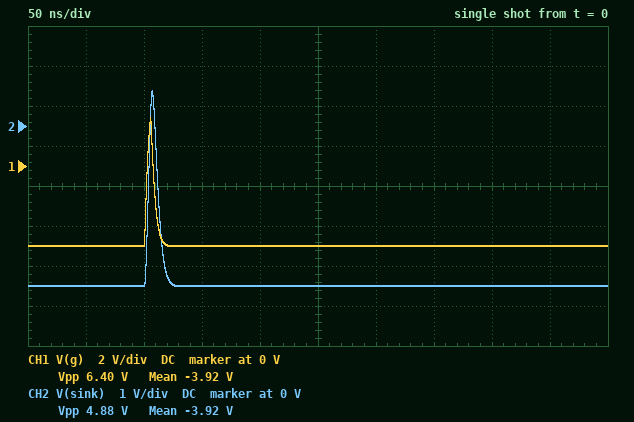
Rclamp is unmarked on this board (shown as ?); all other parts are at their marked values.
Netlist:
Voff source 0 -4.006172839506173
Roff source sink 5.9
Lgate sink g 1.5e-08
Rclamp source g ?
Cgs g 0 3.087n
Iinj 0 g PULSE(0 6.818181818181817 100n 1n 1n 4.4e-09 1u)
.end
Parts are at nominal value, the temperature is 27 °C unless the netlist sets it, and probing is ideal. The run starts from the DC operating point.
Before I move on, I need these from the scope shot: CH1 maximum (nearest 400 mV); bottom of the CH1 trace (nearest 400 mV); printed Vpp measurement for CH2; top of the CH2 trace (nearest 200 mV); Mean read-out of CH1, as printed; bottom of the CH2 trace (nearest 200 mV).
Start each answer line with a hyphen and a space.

- 2.4 V
- -4.0 V
- 4.88 V
- 800 mV
- -3.92 V
- -4.0 V
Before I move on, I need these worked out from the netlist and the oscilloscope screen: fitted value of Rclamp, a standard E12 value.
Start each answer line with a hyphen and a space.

- 1.5 Ω
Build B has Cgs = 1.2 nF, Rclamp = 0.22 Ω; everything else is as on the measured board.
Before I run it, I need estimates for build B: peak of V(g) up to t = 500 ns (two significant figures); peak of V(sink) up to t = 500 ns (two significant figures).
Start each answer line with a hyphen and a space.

- -2.5 V
- -2.8 V
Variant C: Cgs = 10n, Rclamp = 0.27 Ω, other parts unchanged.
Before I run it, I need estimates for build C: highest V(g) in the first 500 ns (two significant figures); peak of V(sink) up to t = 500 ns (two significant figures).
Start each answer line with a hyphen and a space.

- -2.5 V
- -2.8 V
